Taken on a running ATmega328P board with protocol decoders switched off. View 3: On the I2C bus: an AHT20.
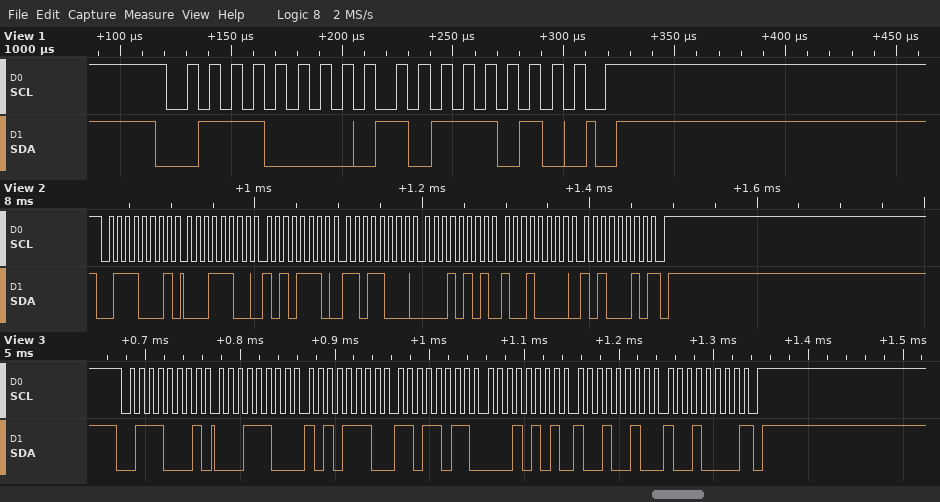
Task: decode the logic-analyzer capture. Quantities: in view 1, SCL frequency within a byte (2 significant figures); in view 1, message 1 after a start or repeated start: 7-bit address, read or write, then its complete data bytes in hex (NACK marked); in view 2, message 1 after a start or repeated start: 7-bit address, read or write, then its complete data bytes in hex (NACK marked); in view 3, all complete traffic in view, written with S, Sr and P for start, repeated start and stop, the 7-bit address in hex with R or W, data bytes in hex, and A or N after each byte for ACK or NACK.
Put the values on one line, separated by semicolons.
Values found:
100 kHz; 0x38 write: BA; 0x38 read: 1C AE D8 15 90 A2 NACK; S 38R A 1C A AE A DB A 15 A 92 A 90 N P
